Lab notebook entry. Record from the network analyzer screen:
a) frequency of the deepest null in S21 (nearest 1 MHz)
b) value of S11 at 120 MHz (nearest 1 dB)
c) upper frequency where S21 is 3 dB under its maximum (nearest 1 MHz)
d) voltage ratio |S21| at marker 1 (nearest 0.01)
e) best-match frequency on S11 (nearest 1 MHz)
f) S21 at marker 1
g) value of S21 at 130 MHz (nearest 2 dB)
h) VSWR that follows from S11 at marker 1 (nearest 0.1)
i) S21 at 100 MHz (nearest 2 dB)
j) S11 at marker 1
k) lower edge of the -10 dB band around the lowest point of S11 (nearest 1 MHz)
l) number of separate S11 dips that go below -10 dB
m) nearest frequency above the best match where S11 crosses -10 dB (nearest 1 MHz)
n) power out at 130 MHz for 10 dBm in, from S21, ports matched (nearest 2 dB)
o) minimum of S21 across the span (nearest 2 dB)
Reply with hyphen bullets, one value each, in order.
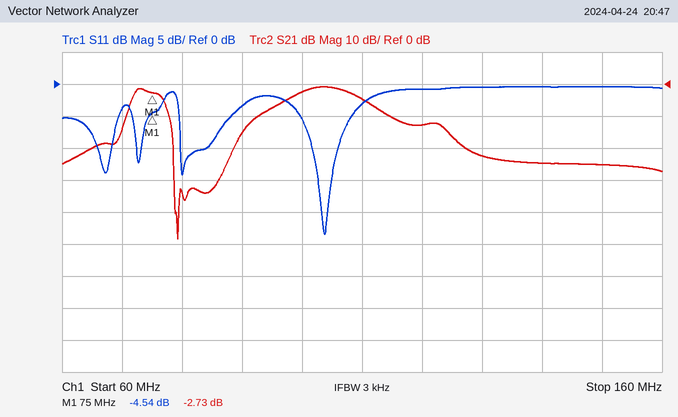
- 79 MHz
- -1 dB
- 109 MHz
- 0.73
- 104 MHz
- -2.73 dB
- -22 dB
- 3.9
- -2 dB
- -4.54 dB
- 102 MHz
- 4
- 106 MHz
- -12 dBm
- -48 dB
